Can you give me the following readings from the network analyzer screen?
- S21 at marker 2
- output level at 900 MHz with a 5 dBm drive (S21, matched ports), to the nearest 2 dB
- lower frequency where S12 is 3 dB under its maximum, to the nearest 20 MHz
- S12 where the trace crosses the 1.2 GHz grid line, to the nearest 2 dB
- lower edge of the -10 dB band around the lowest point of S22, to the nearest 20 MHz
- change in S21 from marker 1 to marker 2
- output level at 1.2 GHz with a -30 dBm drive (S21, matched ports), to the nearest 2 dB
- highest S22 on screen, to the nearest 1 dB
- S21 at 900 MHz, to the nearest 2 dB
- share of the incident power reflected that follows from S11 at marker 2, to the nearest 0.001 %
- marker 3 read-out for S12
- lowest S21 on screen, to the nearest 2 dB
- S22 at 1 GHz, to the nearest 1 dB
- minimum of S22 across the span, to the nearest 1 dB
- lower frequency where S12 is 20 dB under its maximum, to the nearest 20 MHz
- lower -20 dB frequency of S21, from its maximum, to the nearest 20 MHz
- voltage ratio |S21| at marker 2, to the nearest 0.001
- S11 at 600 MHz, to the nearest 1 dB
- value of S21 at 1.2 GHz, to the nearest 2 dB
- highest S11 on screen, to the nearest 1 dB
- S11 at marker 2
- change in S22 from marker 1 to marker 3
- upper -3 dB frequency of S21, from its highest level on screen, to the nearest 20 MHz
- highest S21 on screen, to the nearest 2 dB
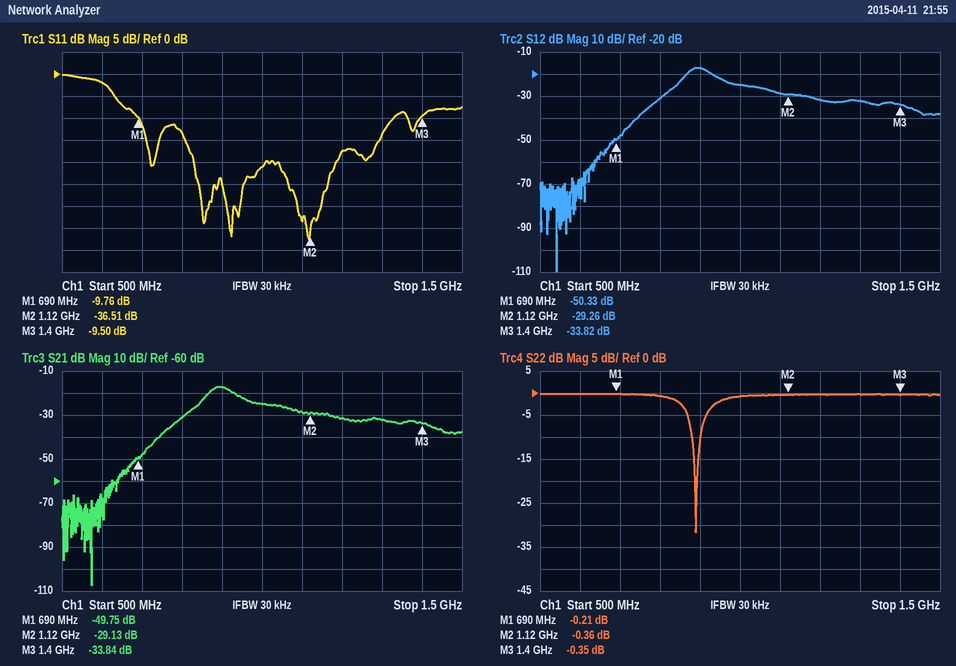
-29.13 dB
-12 dBm
860 MHz
-32 dB
880 MHz
20.62 dB
-62 dBm
0 dB
-18 dB
0.022 %
-33.82 dB
-108 dB
-1 dB
-32 dB
760 MHz
760 MHz
0.035
-2 dB
-32 dB
0 dB
-36.51 dB
-0.14 dB
940 MHz
-18 dB
